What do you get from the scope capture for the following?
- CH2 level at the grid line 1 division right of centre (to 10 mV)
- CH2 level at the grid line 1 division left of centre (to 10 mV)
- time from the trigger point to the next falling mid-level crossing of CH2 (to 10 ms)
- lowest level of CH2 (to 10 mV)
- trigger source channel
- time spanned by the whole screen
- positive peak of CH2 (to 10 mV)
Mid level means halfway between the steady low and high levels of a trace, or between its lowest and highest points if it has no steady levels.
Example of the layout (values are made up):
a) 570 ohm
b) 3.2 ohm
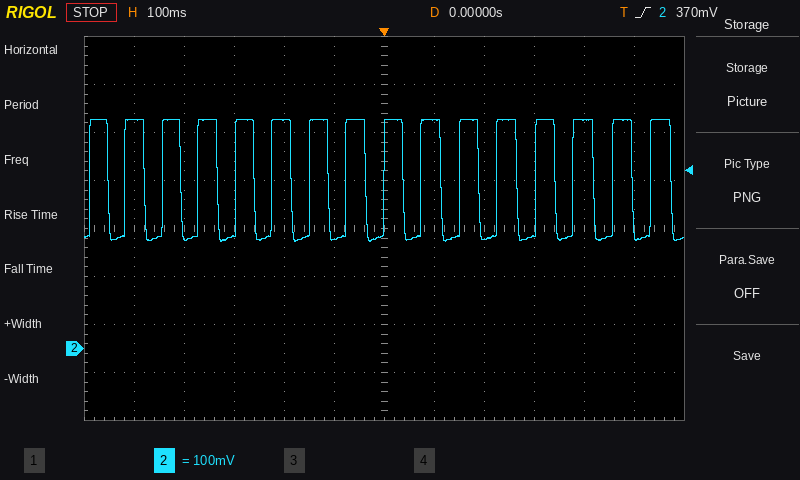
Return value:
a) 480 mV
b) 230 mV
c) 40 ms
d) 220 mV
e) CH2
f) 1.2 s
g) 480 mV
